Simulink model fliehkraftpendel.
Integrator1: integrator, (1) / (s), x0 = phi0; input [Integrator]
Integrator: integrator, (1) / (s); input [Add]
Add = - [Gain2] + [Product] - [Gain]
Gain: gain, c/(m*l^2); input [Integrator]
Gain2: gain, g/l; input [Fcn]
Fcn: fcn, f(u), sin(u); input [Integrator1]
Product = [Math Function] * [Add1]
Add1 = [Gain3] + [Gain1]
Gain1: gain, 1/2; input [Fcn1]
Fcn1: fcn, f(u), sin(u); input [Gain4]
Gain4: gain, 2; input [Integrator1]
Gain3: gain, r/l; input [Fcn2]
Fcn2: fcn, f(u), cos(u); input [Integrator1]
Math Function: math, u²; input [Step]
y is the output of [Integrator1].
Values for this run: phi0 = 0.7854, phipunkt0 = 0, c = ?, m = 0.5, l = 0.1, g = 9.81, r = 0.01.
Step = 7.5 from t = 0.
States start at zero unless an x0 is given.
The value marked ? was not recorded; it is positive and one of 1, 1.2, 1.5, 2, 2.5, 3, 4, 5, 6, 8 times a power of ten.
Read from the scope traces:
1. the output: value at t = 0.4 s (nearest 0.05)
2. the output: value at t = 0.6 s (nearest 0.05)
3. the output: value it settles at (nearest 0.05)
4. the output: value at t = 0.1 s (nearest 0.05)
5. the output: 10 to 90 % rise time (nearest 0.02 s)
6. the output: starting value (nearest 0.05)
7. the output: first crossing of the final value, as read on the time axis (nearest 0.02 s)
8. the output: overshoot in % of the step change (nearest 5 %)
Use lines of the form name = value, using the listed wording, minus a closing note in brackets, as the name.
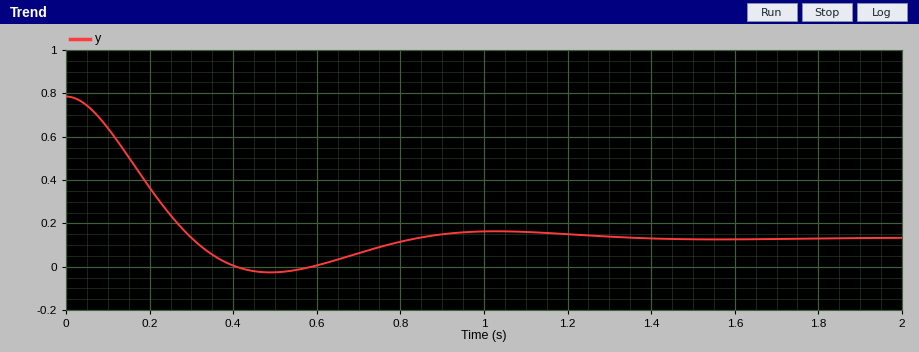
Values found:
the output: value at t = 0.4 s = 0.00
the output: value at t = 0.6 s = 0.00
the output: value it settles at = 0.15
the output: value at t = 0.1 s = 0.65
the output: 10 to 90 % rise time = 0.20 s
the output: starting value = 0.80
the output: first crossing of the final value, as read on the time axis = 0.30 s
the output: overshoot in % of the step change = 25 %
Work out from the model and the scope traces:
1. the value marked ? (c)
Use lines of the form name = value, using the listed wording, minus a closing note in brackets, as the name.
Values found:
the value marked ? = 0.03
